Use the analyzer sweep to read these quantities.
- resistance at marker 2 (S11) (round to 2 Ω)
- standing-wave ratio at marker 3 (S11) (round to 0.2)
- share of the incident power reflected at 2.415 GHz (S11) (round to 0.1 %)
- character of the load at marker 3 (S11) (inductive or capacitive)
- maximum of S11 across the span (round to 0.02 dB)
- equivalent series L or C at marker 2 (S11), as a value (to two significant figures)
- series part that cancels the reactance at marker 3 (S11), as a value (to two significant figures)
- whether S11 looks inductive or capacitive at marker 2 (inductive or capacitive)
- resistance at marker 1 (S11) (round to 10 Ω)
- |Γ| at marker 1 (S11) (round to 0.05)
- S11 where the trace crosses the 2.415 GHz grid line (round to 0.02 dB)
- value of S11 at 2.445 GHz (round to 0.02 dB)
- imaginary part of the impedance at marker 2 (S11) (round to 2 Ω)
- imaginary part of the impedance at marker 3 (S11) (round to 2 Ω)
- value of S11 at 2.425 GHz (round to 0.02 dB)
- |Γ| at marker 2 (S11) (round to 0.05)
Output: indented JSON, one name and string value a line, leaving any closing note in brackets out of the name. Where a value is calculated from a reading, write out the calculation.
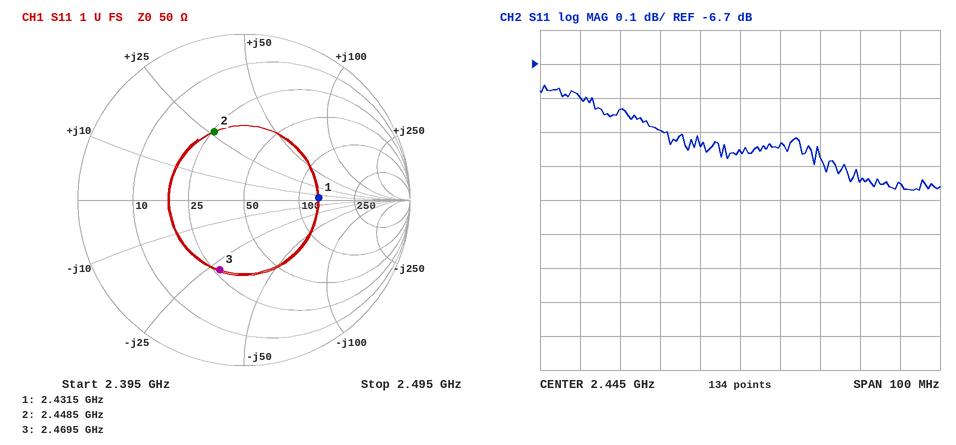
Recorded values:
{
  "resistance at marker 2 (S11)": "26 Ω",
  "standing-wave ratio at marker 3 (S11)": "2.6",
  "share of the incident power reflected at 2.415 GHz (S11)": "10^(-6.84/10) ≈ 20.7 %",
  "character of the load at marker 3 (S11)": "capacitive",
  "maximum of S11 across the span": "-6.76 dB",
  "equivalent series L or C at marker 2 (S11), as a value": "L = 26 Ω/(2π × 2.4485 GHz) ≈ 1.7 nH",
  "series part that cancels the reactance at marker 3 (S11), as a value": "L = 28 Ω/(2π × 2.4695 GHz) ≈ 1.8 nH",
  "whether S11 looks inductive or capacitive at marker 2": "inductive",
  "resistance at marker 1 (S11)": "130 Ω",
  "|Γ| at marker 1 (S11)": "0.45",
  "S11 where the trace crosses the 2.415 GHz grid line": "-6.84 dB",
  "value of S11 at 2.445 GHz": "-6.96 dB",
  "imaginary part of the impedance at marker 2 (S11)": "+26 Ω",
  "imaginary part of the impedance at marker 3 (S11)": "-28 Ω",
  "value of S11 at 2.425 GHz": "-6.90 dB",
  "|Γ| at marker 2 (S11)": "0.45"
}
